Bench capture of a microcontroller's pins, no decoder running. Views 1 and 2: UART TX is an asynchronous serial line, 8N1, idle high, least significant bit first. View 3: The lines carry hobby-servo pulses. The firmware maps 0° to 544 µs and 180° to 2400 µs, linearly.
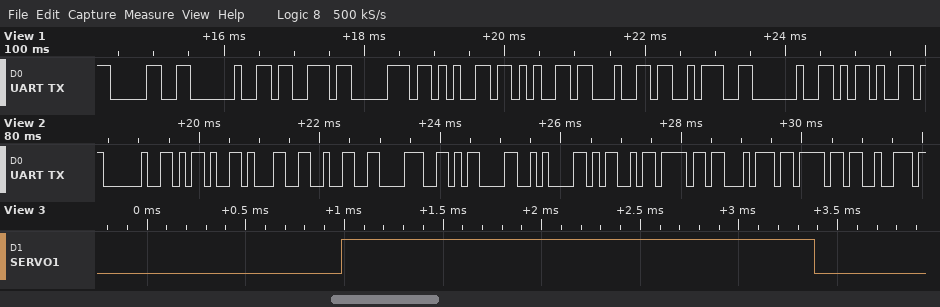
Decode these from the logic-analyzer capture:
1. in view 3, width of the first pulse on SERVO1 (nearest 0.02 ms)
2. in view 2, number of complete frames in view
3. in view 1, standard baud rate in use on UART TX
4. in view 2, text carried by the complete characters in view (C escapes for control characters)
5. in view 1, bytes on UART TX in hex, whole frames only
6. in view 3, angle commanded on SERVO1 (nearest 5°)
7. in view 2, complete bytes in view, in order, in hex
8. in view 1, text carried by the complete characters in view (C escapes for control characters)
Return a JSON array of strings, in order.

["2.40 ms", "12", "9600 baud", "\" -128\\r\\nMotor\"", "30 20 73 70 65 65 64 3A 20 2D", "180°", "0x20 0x2D 0x31 0x32 0x38 0x0D 0x0A 0x4D 0x6F 0x74 0x6F 0x72", "\"0 speed: -\""]
